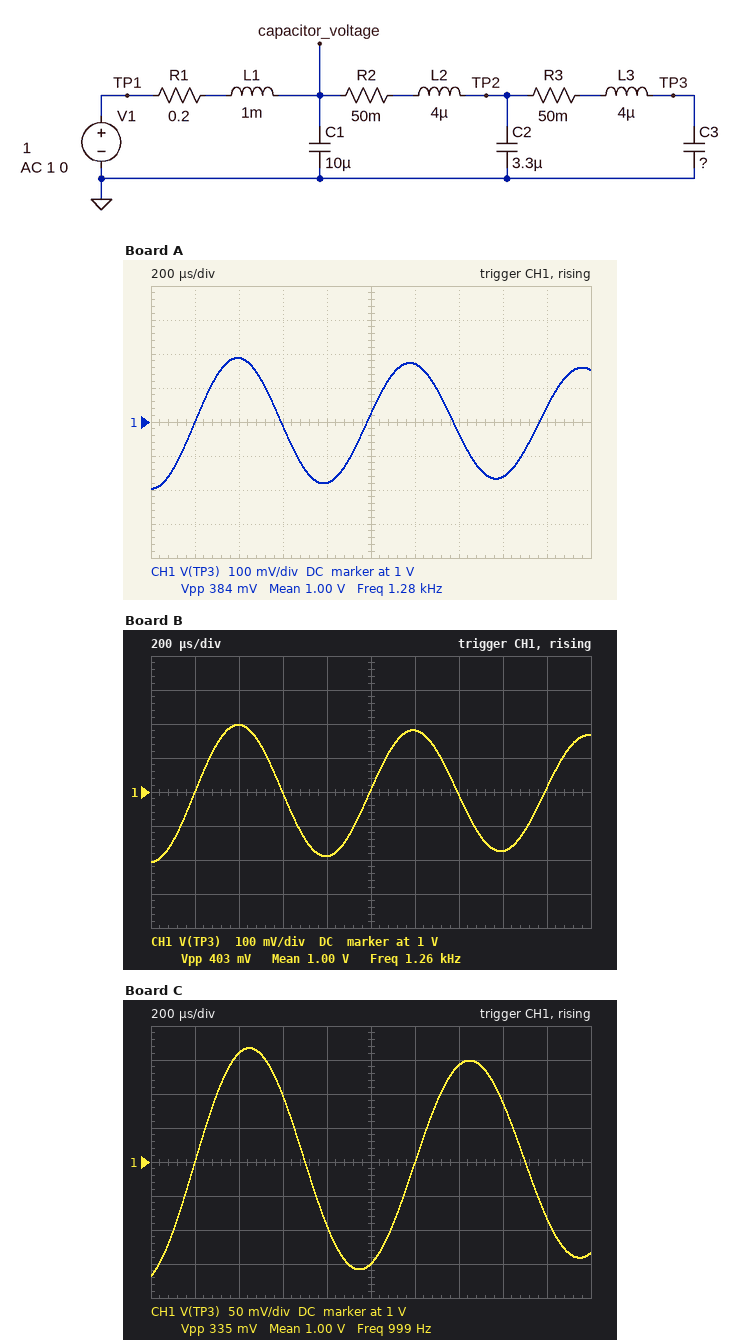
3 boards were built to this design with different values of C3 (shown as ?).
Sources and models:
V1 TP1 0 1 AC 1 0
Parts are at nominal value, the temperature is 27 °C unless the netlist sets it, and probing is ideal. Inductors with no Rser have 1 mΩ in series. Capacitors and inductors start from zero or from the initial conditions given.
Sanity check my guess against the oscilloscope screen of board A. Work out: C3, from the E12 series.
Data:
2.2 µF
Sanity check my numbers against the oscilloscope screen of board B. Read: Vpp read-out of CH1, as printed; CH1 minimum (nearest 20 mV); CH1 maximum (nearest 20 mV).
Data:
403 mV
800 mV
1.20 V
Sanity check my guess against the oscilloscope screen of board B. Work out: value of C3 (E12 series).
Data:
2.7 µF
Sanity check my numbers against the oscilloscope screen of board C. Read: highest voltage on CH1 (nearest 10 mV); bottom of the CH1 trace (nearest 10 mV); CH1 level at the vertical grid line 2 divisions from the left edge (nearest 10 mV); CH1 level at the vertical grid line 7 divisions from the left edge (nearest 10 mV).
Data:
1.17 V
830 mV
1.16 V
1.14 V
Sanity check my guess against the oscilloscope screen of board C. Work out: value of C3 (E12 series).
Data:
12 µF
